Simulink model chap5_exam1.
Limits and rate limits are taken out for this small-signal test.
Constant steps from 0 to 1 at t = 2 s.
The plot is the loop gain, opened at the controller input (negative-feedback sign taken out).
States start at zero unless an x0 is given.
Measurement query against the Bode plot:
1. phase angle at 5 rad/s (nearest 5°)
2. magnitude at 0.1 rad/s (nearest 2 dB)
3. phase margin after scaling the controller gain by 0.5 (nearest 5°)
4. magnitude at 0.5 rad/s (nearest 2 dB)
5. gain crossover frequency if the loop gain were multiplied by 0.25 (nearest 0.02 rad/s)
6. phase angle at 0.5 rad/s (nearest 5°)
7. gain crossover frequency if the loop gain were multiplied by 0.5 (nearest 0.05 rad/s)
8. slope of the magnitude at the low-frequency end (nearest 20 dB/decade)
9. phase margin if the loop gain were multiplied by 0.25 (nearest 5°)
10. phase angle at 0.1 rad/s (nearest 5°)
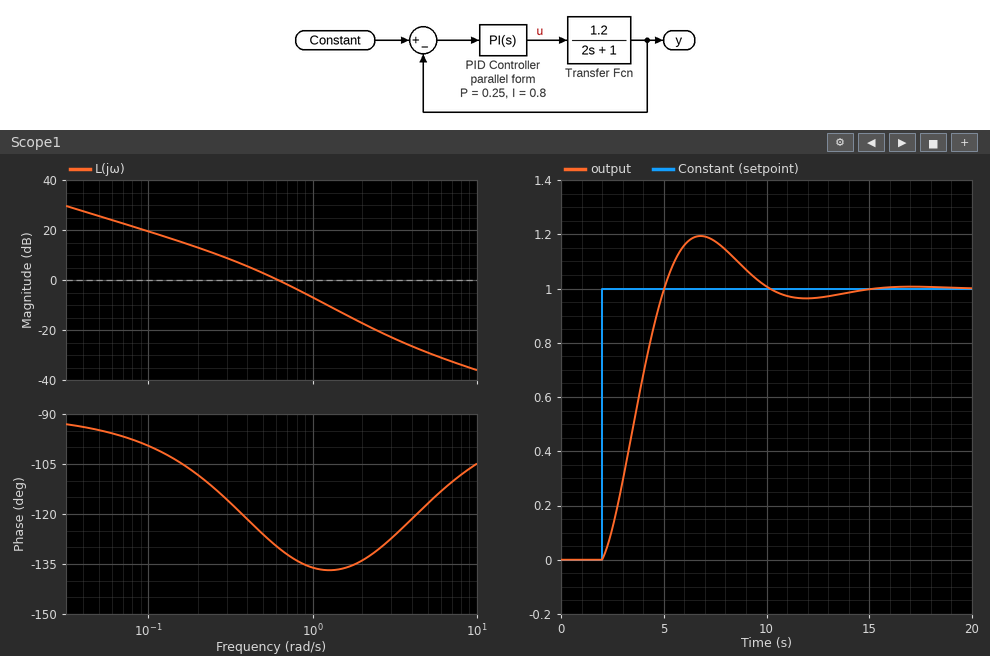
-115°
20 dB
60°
2 dB
0.22 rad/s
-125°
0.40 rad/s
-20 dB/decade
70°
-100°
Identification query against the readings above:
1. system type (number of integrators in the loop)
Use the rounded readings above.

1
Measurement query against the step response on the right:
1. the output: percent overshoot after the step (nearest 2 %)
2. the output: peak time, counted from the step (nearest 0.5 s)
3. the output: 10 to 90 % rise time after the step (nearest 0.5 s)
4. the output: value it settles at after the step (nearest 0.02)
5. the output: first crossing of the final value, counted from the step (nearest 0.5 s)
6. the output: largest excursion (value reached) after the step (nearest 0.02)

20 %
5.0 s
2.0 s
1.00
3.0 s
1.20
